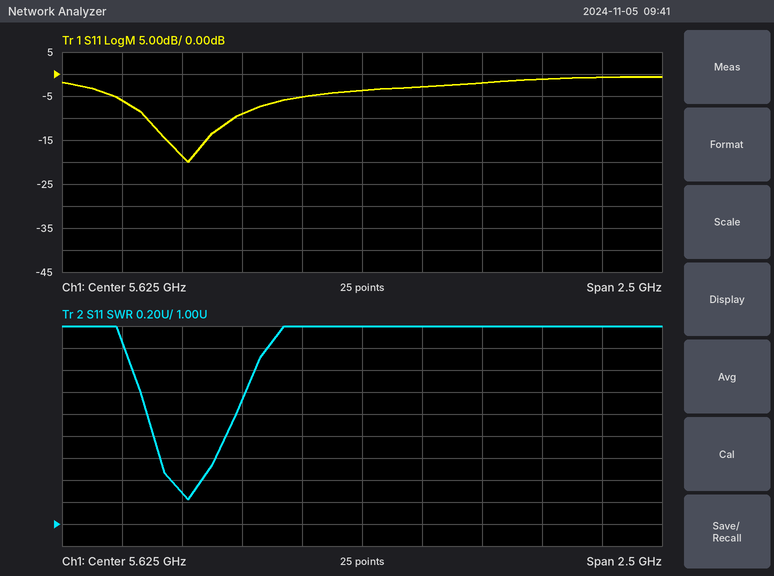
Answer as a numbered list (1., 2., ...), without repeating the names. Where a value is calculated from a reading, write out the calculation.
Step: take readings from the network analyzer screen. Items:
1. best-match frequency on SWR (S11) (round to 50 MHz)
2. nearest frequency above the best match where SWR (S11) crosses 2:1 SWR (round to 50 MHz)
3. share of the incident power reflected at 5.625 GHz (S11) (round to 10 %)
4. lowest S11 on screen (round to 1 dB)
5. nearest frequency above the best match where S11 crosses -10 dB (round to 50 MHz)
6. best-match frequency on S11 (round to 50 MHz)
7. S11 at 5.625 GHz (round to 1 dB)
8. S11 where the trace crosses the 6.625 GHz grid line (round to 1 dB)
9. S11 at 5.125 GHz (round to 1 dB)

1. 4.90 GHz
2. 5.10 GHz
3. 10^(-4/10) ≈ 40 %
4. -20 dB
5. 5.10 GHz
6. 4.90 GHz
7. -4 dB
8. -1 dB
9. -9 dB
